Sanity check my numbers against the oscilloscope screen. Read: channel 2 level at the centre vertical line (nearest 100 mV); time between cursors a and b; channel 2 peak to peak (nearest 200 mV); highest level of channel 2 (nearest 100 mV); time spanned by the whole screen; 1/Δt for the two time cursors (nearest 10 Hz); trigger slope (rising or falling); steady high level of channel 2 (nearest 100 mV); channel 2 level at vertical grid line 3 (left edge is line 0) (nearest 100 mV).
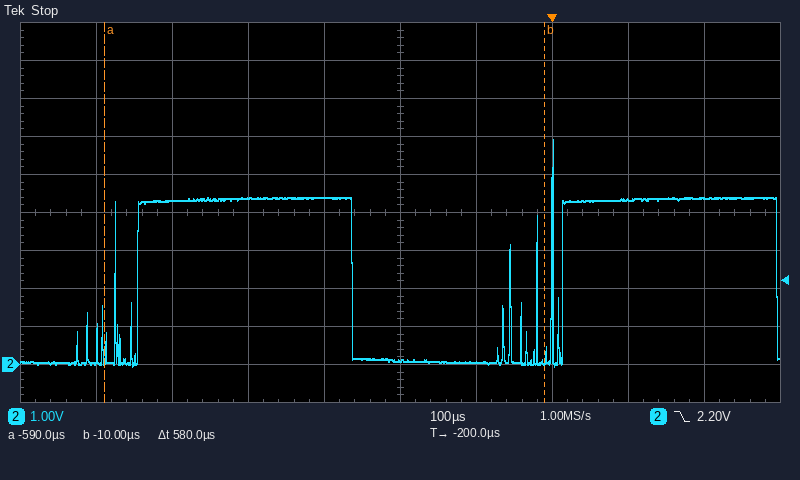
100 mV
580 µs
6.0 V
5.9 V
1 ms
1.72 kHz
falling
4.4 V
4.4 V
